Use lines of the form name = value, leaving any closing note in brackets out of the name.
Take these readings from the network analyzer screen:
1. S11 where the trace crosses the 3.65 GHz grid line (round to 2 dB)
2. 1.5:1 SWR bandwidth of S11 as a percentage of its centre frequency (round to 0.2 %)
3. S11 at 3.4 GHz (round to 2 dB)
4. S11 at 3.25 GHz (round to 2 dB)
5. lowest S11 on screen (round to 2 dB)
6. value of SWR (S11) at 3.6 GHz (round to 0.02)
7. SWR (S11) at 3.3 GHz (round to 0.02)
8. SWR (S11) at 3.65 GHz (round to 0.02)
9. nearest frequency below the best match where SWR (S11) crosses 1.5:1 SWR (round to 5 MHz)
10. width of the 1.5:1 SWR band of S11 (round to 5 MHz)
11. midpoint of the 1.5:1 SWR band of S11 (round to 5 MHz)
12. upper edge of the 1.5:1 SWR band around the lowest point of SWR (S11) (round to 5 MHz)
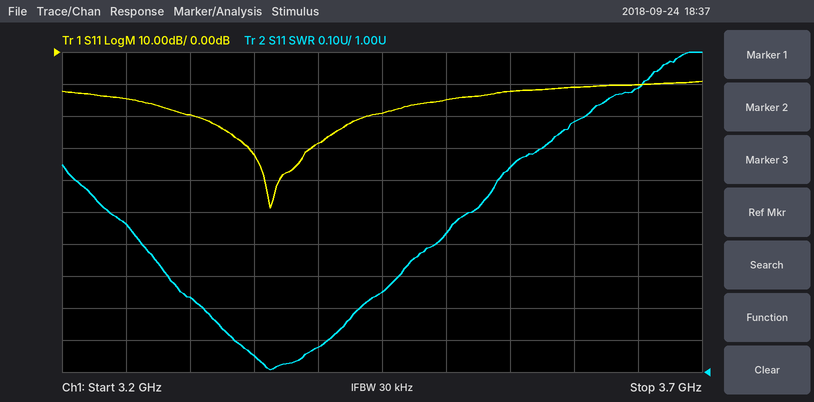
S11 where the trace crosses the 3.65 GHz grid line = -10 dB
1.5:1 SWR bandwidth of S11 as a percentage of its centre frequency = 8.4 %
S11 at 3.4 GHz = -28 dB
S11 at 3.25 GHz = -14 dB
lowest S11 on screen = -48 dB
value of SWR (S11) at 3.6 GHz = 1.78
SWR (S11) at 3.3 GHz = 1.24
SWR (S11) at 3.65 GHz = 1.88
nearest frequency below the best match where SWR (S11) crosses 1.5:1 SWR = 3.235 GHz
width of the 1.5:1 SWR band of S11 = 285 MHz
midpoint of the 1.5:1 SWR band of S11 = 3.380 GHz
upper edge of the 1.5:1 SWR band around the lowest point of SWR (S11) = 3.520 GHz
